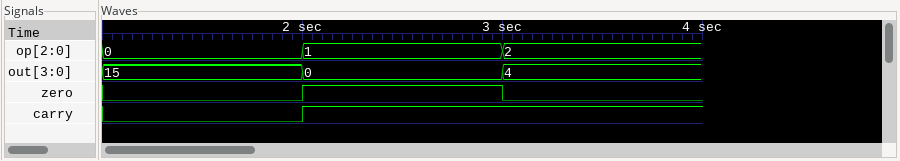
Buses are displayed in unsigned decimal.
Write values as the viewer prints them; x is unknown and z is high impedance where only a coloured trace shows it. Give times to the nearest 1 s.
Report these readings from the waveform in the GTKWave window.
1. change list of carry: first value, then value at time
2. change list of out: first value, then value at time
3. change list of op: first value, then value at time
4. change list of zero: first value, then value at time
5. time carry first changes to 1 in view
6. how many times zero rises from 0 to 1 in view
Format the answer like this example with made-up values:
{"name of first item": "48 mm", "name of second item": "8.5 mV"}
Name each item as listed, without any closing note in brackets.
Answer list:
{"change list of carry: first value, then value at time": "0, 1 at 2 s", "change list of out: first value, then value at time": "15, 0 at 2 s, 4 at 3 s", "change list of op: first value, then value at time": "0, 1 at 2 s, 2 at 3 s", "change list of zero: first value, then value at time": "0, 1 at 2 s, 0 at 3 s", "time carry first changes to 1 in view": "2 s", "how many times zero rises from 0 to 1 in view": "1"}
